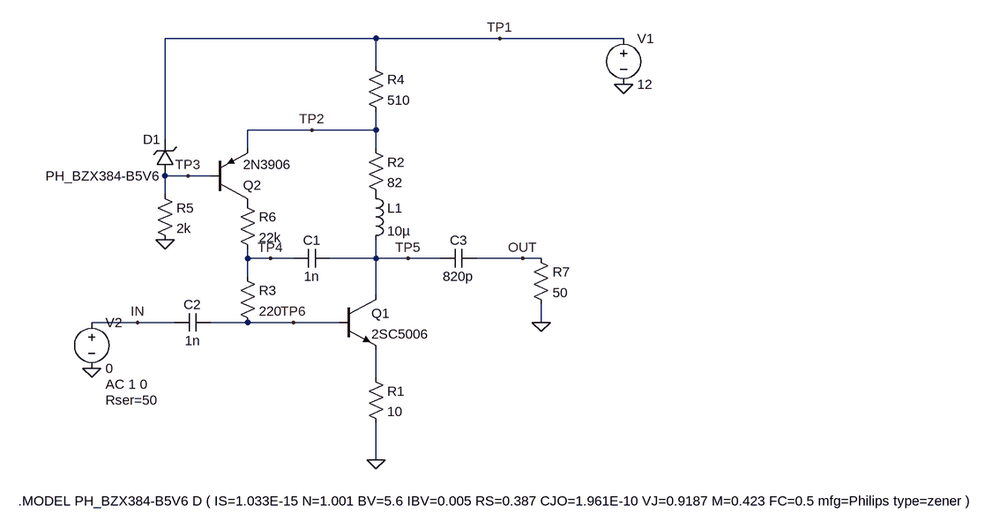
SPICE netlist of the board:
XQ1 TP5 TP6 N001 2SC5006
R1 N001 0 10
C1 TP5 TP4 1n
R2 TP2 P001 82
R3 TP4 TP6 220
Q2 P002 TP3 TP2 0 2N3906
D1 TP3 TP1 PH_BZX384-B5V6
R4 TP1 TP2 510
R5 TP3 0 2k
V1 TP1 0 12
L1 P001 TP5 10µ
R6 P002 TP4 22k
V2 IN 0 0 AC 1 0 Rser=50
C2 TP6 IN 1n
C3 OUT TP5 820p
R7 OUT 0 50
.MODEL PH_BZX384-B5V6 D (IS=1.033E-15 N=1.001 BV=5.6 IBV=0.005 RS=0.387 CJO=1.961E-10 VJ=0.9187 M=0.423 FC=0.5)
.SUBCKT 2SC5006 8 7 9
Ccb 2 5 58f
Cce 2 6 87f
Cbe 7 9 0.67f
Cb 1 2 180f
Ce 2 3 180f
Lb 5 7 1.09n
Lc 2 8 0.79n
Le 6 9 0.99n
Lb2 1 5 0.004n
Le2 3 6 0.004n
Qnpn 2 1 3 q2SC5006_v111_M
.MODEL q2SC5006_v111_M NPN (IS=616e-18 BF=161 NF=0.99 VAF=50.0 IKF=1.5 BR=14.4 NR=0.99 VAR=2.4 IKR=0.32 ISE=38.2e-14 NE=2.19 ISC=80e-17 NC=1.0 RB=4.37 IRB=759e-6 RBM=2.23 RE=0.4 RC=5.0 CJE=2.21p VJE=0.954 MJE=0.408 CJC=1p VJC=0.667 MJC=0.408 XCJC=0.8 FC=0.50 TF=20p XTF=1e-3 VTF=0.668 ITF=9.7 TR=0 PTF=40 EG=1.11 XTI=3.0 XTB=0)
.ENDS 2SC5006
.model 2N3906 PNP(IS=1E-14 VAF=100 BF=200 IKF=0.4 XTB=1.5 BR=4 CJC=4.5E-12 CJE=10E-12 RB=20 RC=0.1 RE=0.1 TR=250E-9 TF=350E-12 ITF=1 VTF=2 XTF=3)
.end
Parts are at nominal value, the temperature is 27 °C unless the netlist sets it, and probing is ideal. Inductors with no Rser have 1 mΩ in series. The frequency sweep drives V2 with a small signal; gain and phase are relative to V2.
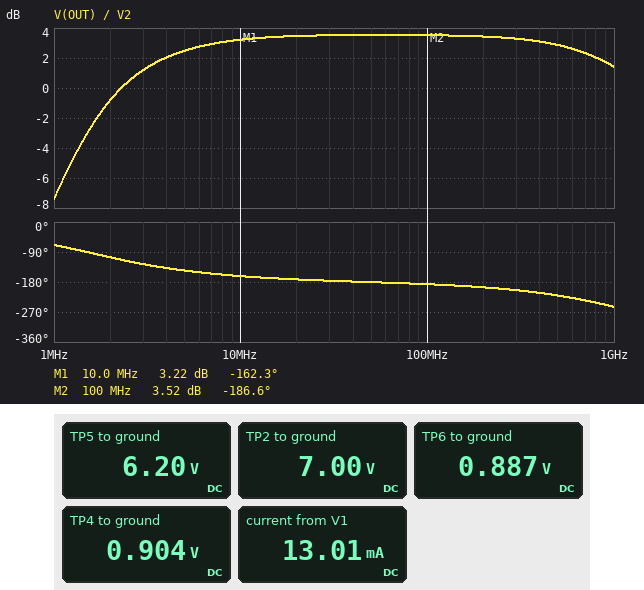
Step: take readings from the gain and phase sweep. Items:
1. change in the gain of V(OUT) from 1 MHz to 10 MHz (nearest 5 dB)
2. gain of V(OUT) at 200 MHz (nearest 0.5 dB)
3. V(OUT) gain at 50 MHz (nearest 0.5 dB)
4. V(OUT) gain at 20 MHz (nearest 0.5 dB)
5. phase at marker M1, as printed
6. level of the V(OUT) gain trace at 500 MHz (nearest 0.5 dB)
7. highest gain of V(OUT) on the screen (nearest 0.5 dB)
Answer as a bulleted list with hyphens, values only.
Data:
- 10 dB
- 3.5 dB
- 3.5 dB
- 3.5 dB
- -162.3 deg
- 3.0 dB
- 3.5 dB
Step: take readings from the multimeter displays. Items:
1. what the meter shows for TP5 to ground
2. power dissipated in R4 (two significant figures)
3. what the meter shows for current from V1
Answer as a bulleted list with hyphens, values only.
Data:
- 6.20 V
- 49 mW
- 13.01 mA
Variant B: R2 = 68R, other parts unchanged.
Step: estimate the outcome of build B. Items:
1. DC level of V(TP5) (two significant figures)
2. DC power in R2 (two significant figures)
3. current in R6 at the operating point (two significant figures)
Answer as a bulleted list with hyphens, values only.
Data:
- 6.3 V
- 6.4 mW
- 78 µA
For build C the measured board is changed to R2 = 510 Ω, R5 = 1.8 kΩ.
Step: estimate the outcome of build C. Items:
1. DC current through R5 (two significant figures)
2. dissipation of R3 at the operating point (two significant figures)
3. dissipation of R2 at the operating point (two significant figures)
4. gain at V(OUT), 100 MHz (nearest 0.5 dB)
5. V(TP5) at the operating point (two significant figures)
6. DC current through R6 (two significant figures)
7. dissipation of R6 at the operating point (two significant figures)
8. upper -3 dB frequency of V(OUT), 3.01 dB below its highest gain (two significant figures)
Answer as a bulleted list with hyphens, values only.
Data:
- 3.6 mA
- 1.7 µW
- 48 mW
- 3.5 dB
- 2.0 V
- 88 µA
- 170 µW
- 1.0 GHz
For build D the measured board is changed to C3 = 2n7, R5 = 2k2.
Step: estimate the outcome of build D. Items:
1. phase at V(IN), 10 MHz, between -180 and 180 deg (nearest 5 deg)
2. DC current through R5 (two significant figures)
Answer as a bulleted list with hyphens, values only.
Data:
- -10 deg
- 2.9 mA
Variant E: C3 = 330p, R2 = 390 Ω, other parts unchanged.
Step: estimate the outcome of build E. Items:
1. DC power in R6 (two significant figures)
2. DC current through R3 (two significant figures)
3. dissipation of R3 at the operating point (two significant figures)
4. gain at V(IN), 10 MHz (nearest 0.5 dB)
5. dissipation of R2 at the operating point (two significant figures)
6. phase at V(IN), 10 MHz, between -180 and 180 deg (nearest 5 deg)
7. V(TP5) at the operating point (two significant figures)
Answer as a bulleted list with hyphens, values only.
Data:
- 160 µW
- 85 µA
- 1.6 µW
- -6.5 dB
- 37 mW
- 0 deg
- 3.2 V
